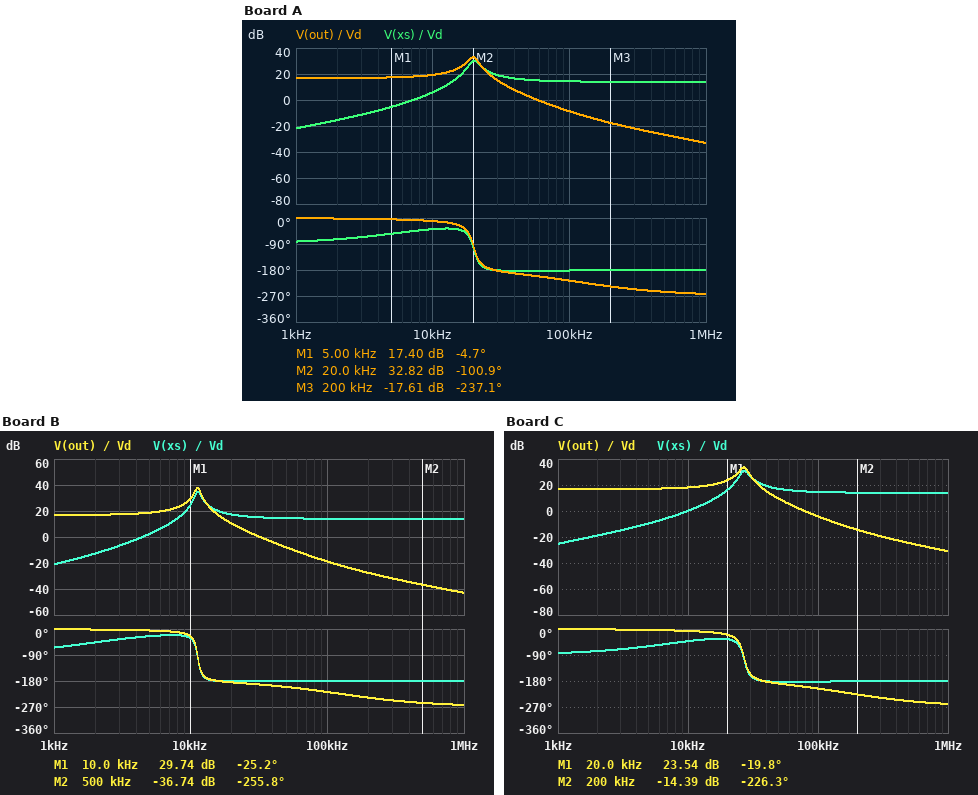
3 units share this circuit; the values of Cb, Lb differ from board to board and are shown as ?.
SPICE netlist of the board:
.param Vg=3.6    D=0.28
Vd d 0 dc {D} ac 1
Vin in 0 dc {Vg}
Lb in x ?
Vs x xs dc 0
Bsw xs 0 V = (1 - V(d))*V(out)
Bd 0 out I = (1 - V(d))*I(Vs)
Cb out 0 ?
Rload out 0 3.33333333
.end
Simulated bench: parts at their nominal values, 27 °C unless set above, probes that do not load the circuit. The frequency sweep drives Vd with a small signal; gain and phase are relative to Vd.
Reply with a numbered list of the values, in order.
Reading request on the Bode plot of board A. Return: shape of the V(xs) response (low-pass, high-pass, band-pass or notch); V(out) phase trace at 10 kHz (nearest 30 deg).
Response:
1. high-pass
2. 0 deg
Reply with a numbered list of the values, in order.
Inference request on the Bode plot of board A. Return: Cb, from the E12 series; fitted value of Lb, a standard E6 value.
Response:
1. 15 µF
2. 2.2 µH
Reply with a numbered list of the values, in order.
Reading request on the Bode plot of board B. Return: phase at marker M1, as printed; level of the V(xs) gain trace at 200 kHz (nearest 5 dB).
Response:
1. -25.2 deg
2. 15 dB
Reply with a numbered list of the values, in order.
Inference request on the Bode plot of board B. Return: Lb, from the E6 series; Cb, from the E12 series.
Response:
1. 2.2 µH
2. 47 µF
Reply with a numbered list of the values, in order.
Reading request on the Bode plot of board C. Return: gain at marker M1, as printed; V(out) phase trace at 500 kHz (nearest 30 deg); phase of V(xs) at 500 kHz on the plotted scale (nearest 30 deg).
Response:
1. 23.54 dB
2. -240 deg
3. -180 deg
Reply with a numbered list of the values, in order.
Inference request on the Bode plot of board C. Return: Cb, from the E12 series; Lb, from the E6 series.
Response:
1. 12 µF
2. 1.5 µH
